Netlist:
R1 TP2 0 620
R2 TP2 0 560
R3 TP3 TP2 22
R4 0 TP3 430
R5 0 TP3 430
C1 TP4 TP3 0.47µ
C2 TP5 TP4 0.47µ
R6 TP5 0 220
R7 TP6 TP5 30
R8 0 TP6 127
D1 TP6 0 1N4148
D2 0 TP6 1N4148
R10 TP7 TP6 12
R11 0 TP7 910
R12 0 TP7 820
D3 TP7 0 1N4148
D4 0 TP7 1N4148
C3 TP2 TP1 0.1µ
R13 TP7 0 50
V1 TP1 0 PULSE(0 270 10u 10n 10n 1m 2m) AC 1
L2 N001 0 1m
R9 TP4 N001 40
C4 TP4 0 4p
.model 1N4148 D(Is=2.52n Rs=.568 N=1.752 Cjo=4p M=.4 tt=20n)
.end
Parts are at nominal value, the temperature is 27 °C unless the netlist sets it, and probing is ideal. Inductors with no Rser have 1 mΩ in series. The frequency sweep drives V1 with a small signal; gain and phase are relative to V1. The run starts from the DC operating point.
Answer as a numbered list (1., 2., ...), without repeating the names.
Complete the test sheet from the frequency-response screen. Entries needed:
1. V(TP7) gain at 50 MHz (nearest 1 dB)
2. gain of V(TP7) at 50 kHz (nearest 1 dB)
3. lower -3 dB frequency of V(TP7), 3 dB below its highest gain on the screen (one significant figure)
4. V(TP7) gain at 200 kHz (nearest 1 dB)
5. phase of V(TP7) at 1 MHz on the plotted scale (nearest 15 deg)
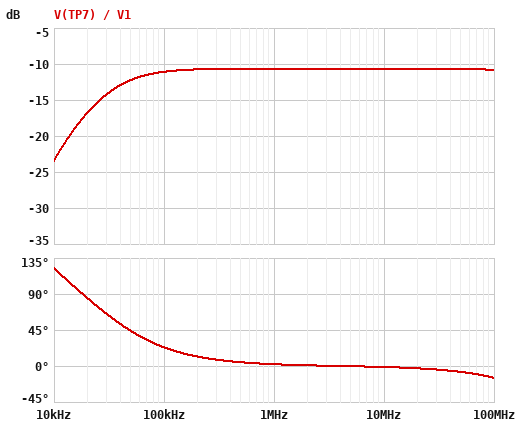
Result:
1. -11 dB
2. -12 dB
3. 30 kHz
4. -11 dB
5. 0 deg
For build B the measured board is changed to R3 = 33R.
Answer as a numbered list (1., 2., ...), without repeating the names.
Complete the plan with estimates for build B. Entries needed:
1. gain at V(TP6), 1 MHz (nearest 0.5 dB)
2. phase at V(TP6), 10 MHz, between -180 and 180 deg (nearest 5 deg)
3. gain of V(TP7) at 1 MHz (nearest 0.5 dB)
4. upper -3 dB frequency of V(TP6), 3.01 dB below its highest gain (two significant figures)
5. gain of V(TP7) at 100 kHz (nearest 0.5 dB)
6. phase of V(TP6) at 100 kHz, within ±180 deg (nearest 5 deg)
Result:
1. -10.0 dB
2. 0 deg
3. -12.0 dB
4. 450 MHz
5. -12.5 dB
6. 20 deg
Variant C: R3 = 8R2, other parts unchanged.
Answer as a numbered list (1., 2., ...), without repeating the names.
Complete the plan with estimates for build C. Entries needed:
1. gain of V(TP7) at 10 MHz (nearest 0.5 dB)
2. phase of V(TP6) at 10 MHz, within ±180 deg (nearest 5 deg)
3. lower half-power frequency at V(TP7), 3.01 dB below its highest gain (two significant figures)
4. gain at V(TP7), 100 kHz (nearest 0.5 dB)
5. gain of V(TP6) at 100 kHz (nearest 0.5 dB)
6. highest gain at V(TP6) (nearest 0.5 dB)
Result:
1. -8.5 dB
2. 0 deg
3. 41 kHz
4. -9.0 dB
5. -7.0 dB
6. -6.5 dB
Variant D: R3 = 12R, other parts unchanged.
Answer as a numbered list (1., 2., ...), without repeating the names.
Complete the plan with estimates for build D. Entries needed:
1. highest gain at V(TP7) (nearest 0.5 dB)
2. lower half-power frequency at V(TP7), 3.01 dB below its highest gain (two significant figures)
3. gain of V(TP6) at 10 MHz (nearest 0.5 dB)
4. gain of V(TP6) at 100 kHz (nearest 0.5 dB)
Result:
1. -9.0 dB
2. 39 kHz
3. -7.0 dB
4. -7.5 dB
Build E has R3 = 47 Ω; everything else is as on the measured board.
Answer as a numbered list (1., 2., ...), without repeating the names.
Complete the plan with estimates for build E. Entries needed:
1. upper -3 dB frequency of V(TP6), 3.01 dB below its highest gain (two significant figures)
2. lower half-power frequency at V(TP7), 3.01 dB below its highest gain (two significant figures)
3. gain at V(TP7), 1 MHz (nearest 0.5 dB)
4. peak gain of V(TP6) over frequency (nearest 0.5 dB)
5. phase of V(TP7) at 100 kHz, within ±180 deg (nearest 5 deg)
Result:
1. 420 MHz
2. 27 kHz
3. -13.5 dB
4. -11.5 dB
5. 20 deg
